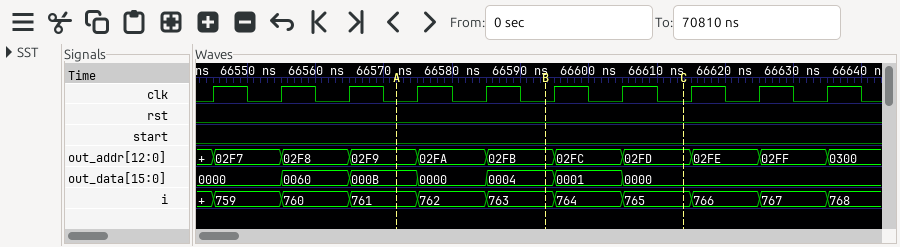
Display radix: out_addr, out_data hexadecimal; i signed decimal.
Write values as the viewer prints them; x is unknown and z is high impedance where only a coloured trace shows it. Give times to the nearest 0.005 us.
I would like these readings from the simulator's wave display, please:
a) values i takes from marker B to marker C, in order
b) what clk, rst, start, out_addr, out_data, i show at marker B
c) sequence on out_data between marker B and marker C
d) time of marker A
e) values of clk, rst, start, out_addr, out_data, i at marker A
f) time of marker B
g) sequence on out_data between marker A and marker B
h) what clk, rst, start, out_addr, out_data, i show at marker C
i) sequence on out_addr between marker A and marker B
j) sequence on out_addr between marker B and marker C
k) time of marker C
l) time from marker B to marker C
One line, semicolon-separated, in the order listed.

763, 764, 765; clk=0, rst=0, start=0, out_addr=02FB, out_data=0004, i=763; 0004, 0001, 0000; 66.57 us; clk=0, rst=0, start=0, out_addr=02F9, out_data=000B, i=761; 66.595 us; 000B, 0000, 0004; clk=0, rst=0, start=0, out_addr=02FD, out_data=0000, i=765; 02F9, 02FA, 02FB; 02FB, 02FC, 02FD; 66.615 us; 0.02 us
